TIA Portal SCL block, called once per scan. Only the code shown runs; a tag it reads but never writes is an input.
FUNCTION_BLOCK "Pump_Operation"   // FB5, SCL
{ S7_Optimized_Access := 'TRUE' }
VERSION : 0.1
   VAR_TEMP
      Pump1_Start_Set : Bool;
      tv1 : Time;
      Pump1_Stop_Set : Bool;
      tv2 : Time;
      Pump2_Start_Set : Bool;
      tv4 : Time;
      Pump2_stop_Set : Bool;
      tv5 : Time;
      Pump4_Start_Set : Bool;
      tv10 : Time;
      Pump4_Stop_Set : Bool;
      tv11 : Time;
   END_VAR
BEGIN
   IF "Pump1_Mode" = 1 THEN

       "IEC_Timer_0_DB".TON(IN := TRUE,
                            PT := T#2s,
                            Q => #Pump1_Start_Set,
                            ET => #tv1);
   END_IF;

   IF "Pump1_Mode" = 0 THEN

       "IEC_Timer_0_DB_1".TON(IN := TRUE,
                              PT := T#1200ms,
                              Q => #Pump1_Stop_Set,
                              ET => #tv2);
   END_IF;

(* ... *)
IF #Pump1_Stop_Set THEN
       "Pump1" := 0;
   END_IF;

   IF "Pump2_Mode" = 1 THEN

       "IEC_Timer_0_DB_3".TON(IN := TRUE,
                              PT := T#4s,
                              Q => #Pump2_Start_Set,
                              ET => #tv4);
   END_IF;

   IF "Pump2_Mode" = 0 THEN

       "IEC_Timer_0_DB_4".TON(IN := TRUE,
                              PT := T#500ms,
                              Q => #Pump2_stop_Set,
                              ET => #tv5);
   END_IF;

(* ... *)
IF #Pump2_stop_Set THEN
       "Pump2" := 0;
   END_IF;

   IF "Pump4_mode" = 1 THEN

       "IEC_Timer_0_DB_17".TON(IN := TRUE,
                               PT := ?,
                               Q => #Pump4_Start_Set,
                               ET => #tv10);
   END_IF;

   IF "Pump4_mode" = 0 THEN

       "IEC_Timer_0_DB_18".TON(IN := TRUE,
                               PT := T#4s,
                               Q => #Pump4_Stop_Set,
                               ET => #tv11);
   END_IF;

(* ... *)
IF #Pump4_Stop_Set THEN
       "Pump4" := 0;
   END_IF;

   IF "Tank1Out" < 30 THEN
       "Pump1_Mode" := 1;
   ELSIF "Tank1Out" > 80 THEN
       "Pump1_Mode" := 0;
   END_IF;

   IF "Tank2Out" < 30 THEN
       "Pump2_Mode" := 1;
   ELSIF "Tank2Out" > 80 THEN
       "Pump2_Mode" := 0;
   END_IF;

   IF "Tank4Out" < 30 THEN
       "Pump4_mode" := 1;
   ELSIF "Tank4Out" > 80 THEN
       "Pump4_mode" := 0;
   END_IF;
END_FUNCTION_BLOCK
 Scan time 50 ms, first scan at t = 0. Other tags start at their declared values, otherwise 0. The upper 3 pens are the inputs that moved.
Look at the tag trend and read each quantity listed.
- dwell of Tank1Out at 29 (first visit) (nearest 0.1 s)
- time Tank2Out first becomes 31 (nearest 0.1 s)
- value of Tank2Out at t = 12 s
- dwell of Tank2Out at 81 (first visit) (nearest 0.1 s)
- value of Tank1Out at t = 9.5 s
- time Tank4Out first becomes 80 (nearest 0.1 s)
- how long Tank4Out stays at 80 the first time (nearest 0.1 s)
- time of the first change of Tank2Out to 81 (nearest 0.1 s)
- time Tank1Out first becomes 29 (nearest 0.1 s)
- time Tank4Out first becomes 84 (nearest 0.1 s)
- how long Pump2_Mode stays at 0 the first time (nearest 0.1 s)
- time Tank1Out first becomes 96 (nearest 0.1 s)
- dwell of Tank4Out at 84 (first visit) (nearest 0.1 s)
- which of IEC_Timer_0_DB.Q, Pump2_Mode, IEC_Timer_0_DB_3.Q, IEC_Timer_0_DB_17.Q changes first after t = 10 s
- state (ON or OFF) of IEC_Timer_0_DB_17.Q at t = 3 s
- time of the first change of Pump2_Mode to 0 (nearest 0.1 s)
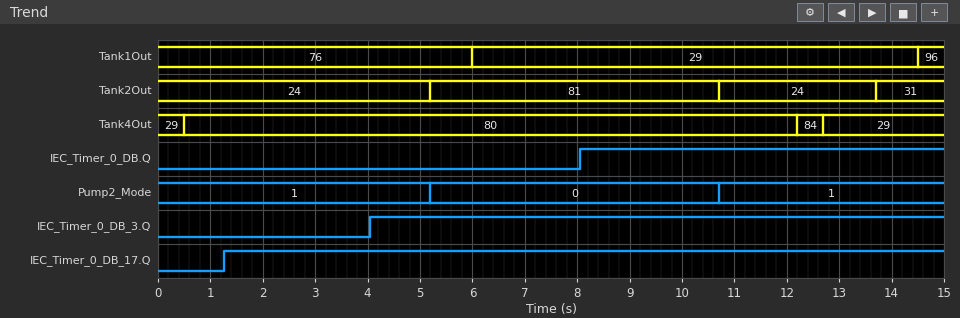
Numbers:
8.5 s
13.7 s
24
5.5 s
29
0.5 s
11.7 s
5.2 s
6.0 s
12.2 s
5.5 s
14.5 s
0.5 s
Pump2_Mode
ON
5.2 s
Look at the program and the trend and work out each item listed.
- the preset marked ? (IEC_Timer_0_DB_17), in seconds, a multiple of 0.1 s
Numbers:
1.2 s
